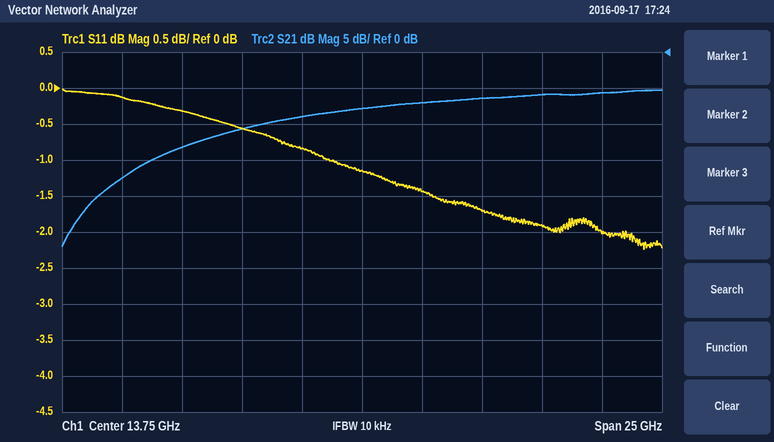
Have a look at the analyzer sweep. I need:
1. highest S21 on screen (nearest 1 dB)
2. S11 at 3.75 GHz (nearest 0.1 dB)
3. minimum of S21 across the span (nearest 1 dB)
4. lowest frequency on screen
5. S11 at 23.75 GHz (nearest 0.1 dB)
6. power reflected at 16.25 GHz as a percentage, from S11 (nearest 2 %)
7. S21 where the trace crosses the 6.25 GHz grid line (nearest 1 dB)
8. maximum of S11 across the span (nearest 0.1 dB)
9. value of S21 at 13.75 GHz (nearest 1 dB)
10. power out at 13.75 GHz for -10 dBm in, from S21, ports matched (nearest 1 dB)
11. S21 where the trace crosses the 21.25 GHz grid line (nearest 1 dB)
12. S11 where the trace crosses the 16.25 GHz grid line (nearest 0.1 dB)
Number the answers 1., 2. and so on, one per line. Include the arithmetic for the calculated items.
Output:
1. -5 dB
2. -0.1 dB
3. -27 dB
4. 1.25 GHz
5. -2.0 dB
6. 10^(-1.4/10) ≈ 72 %
7. -13 dB
8. 0.0 dB
9. -8 dB
10. -10 dBm + (-8 dB) = -18 dBm
11. -6 dB
12. -1.4 dB
